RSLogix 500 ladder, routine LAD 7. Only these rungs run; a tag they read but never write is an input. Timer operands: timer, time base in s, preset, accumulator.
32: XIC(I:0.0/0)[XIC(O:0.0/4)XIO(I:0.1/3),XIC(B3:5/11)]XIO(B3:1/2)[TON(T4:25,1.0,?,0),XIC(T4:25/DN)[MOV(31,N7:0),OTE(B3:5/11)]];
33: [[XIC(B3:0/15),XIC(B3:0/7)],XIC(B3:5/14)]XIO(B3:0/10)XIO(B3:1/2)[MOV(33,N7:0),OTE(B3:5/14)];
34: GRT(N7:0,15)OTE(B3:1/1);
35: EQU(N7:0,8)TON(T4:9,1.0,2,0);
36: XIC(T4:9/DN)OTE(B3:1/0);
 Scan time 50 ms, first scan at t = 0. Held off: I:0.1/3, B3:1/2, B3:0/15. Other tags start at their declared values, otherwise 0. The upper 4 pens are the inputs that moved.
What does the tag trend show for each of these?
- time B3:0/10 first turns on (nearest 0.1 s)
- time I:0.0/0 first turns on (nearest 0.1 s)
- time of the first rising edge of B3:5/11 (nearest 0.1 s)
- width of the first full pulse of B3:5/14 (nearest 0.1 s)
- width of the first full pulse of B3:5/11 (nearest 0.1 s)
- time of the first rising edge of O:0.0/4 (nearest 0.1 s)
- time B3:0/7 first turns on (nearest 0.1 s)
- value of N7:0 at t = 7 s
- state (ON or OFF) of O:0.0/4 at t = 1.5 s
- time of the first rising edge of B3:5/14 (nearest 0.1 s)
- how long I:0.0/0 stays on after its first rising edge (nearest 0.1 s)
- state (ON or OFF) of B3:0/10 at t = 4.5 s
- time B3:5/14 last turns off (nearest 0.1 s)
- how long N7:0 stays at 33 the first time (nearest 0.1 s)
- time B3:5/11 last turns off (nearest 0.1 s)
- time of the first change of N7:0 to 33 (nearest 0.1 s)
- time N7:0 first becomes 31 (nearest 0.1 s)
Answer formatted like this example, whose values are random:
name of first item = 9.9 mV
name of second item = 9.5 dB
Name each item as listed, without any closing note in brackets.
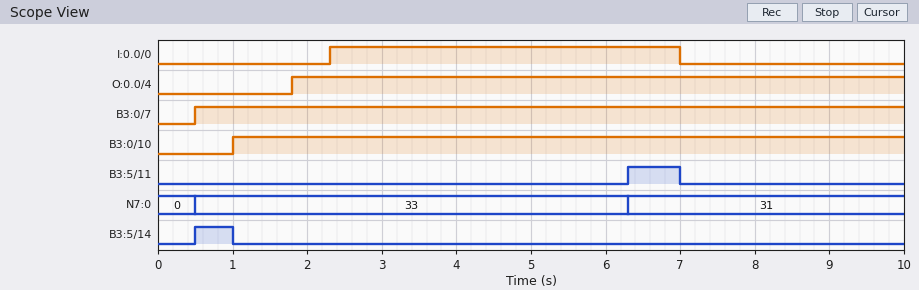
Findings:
time B3:0/10 first turns on = 1.0 s
time I:0.0/0 first turns on = 2.3 s
time of the first rising edge of B3:5/11 = 6.3 s
width of the first full pulse of B3:5/14 = 0.5 s
width of the first full pulse of B3:5/11 = 0.7 s
time of the first rising edge of O:0.0/4 = 1.8 s
time B3:0/7 first turns on = 0.5 s
value of N7:0 at t = 7 s = 31
state (ON or OFF) of O:0.0/4 at t = 1.5 s = OFF
time of the first rising edge of B3:5/14 = 0.5 s
how long I:0.0/0 stays on after its first rising edge = 4.7 s
state (ON or OFF) of B3:0/10 at t = 4.5 s = ON
time B3:5/14 last turns off = 1.0 s
how long N7:0 stays at 33 the first time = 5.8 s
time B3:5/11 last turns off = 7.0 s
time of the first change of N7:0 to 33 = 0.5 s
time N7:0 first becomes 31 = 6.3 s
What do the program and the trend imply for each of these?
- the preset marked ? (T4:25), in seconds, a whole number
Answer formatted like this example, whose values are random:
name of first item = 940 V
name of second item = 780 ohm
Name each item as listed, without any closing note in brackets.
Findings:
the preset marked ? (T4:25), in seconds, a whole number = 4 s
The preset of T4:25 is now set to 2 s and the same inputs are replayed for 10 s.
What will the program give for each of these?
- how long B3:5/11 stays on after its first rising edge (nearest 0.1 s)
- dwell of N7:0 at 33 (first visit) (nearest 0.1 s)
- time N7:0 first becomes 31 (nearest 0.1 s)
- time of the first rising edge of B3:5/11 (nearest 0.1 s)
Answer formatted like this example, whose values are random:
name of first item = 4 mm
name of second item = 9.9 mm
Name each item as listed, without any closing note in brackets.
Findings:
how long B3:5/11 stays on after its first rising edge = 2.7 s
dwell of N7:0 at 33 (first visit) = 3.8 s
time N7:0 first becomes 31 = 4.3 s
time of the first rising edge of B3:5/11 = 4.3 s
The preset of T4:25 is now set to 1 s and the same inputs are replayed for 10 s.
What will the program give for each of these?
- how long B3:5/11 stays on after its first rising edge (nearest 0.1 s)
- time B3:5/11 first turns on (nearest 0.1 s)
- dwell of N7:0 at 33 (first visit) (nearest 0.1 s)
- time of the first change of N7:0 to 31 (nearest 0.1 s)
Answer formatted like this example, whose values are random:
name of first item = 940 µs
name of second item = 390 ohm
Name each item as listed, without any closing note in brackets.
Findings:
how long B3:5/11 stays on after its first rising edge = 3.7 s
time B3:5/11 first turns on = 3.3 s
dwell of N7:0 at 33 (first visit) = 2.8 s
time of the first change of N7:0 to 31 = 3.3 s
